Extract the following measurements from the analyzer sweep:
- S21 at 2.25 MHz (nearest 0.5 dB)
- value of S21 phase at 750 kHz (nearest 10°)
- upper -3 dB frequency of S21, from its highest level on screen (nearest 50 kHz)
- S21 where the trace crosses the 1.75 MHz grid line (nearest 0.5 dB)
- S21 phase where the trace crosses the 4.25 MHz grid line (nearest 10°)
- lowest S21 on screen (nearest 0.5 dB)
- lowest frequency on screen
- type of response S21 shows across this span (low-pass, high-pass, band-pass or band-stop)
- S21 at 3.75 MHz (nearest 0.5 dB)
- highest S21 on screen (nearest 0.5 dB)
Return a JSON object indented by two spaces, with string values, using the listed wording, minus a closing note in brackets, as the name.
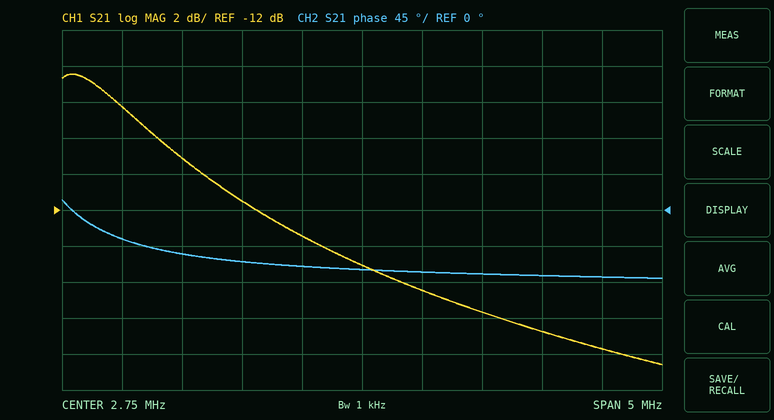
{
  "S21 at 2.25 MHz": "-13.5 dB",
  "value of S21 phase at 750 kHz": "-40°",
  "upper -3 dB frequency of S21, from its highest level on screen": "950 kHz",
  "S21 where the trace crosses the 1.75 MHz grid line": "-11.5 dB",
  "S21 phase where the trace crosses the 4.25 MHz grid line": "-80°",
  "lowest S21 on screen": "-20.5 dB",
  "lowest frequency on screen": "250 kHz",
  "type of response S21 shows across this span": "low-pass",
  "S21 at 3.75 MHz": "-17.5 dB",
  "highest S21 on screen": "-4.5 dB"
}
